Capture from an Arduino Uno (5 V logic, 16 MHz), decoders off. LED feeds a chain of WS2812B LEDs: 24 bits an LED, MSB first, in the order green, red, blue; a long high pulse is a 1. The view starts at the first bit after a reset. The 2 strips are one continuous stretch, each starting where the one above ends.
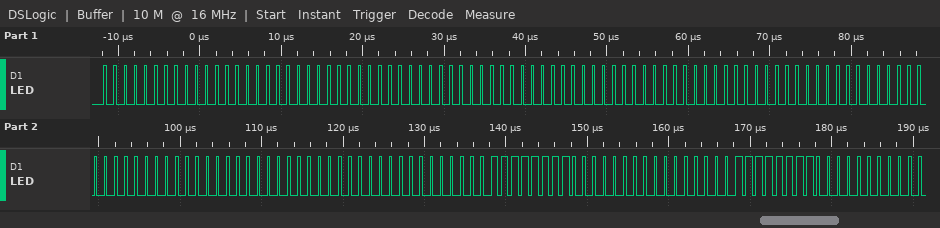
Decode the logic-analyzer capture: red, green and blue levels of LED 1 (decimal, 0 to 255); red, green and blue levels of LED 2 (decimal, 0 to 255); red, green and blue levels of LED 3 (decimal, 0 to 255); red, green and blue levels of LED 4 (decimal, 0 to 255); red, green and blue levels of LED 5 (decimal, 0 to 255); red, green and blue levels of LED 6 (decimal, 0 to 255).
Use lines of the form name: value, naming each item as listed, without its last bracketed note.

red, green and blue levels of LED 1: 0, 0, 0
red, green and blue levels of LED 2: 0, 0, 0
red, green and blue levels of LED 3: 0, 0, 0
red, green and blue levels of LED 4: 0, 0, 0
red, green and blue levels of LED 5: 0, 0, 0
red, green and blue levels of LED 6: 0, 255, 0
